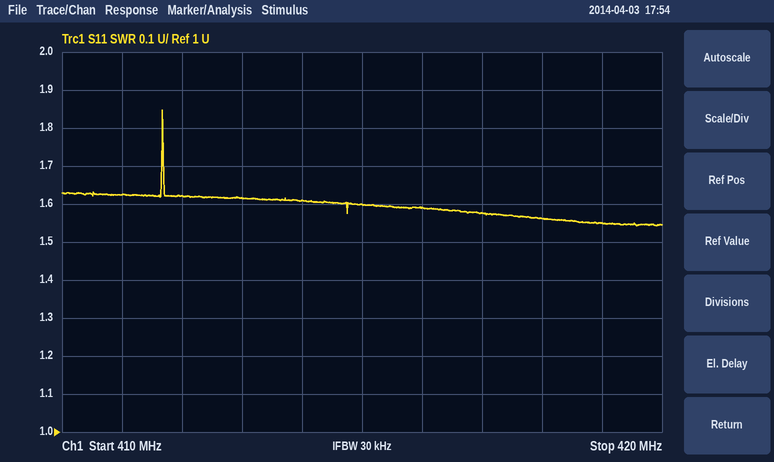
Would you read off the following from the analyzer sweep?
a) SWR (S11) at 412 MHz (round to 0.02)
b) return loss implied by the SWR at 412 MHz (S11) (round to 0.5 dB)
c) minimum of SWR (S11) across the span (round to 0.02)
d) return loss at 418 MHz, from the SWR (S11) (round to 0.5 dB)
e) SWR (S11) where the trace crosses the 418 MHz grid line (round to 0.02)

1.62
12.5 dB
1.54
13.0 dB
1.56
